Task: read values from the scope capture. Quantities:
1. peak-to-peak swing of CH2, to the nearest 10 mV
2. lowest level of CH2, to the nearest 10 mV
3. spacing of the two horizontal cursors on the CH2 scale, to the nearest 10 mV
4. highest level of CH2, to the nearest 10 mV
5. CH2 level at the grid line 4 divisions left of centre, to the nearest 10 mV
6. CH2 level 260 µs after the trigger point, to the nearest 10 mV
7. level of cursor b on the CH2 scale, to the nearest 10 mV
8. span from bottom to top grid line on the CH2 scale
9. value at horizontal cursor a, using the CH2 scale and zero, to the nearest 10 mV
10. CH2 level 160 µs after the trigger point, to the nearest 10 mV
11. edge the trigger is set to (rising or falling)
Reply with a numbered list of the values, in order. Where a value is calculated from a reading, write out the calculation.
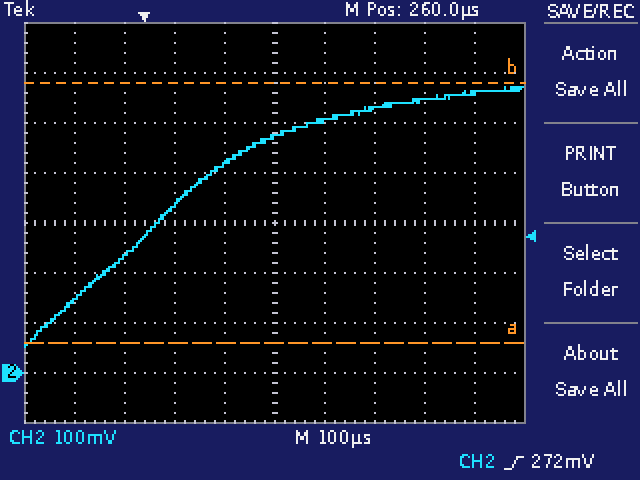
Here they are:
1. 570 mV − (50 mV) = 520 mV
2. 50 mV
3. 520 mV
4. 570 mV
5. 150 mV
6. 470 mV
7. 580 mV
8. 800 mV
9. 60 mV
10. 420 mV
11. rising
